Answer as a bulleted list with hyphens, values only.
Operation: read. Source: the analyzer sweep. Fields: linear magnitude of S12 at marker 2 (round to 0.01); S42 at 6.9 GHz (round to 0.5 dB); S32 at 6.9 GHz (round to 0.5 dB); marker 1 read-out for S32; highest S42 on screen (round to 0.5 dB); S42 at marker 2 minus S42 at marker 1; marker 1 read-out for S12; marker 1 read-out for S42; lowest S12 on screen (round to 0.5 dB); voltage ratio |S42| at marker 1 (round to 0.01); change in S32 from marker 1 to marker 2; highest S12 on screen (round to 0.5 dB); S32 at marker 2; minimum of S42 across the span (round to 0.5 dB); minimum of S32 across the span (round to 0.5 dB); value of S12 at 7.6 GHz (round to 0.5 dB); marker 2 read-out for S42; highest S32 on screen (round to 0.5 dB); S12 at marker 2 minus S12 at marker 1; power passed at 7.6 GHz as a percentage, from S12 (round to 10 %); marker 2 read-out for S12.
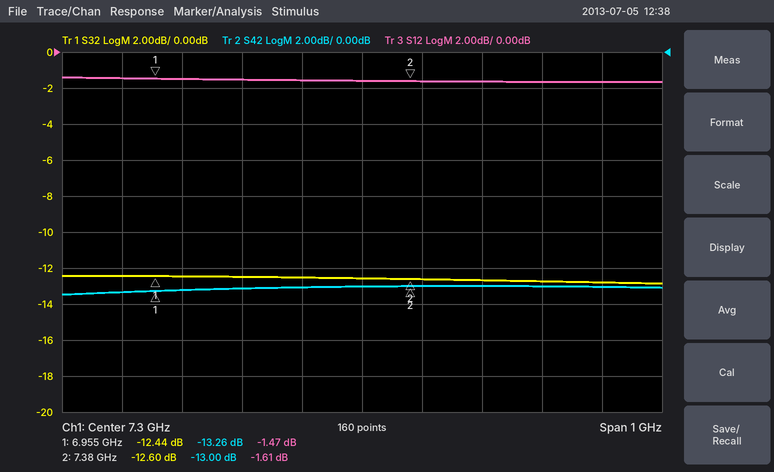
- 0.83
- -13.5 dB
- -12.5 dB
- -12.44 dB
- -13.0 dB
- 0.26 dB
- -1.47 dB
- -13.26 dB
- -1.5 dB
- 0.22
- -0.16 dB
- -1.5 dB
- -12.60 dB
- -13.5 dB
- -13.0 dB
- -1.5 dB
- -13.00 dB
- -12.5 dB
- -0.14 dB
- 70 %
- -1.61 dB
